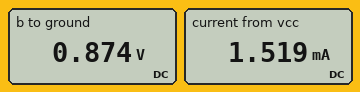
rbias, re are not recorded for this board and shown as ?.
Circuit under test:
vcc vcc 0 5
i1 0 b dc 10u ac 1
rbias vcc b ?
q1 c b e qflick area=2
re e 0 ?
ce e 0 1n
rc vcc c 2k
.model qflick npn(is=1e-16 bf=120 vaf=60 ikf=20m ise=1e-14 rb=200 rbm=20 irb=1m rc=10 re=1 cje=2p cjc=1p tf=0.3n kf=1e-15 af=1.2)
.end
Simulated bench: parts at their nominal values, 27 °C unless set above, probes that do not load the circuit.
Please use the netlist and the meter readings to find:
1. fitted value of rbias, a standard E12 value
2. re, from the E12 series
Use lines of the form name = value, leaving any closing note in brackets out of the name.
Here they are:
fitted value of rbias, a standard E12 value = 390 kΩ
re, from the E12 series = 68 Ω
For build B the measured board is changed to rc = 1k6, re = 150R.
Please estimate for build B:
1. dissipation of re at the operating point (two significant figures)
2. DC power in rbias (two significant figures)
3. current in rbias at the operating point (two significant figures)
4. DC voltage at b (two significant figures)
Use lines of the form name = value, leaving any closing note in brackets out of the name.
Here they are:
dissipation of re at the operating point = 340 µW
DC power in rbias = 41 µW
current in rbias at the operating point = 10 µA
DC voltage at b = 1.0 V
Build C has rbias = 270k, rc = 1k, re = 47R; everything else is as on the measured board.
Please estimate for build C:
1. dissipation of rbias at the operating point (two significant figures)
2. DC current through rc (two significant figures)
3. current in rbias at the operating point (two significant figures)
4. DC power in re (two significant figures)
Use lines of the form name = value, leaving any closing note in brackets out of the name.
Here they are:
dissipation of rbias at the operating point = 63 µW
DC current through rc = 1.9 mA
current in rbias at the operating point = 15 µA
DC power in re = 180 µW
